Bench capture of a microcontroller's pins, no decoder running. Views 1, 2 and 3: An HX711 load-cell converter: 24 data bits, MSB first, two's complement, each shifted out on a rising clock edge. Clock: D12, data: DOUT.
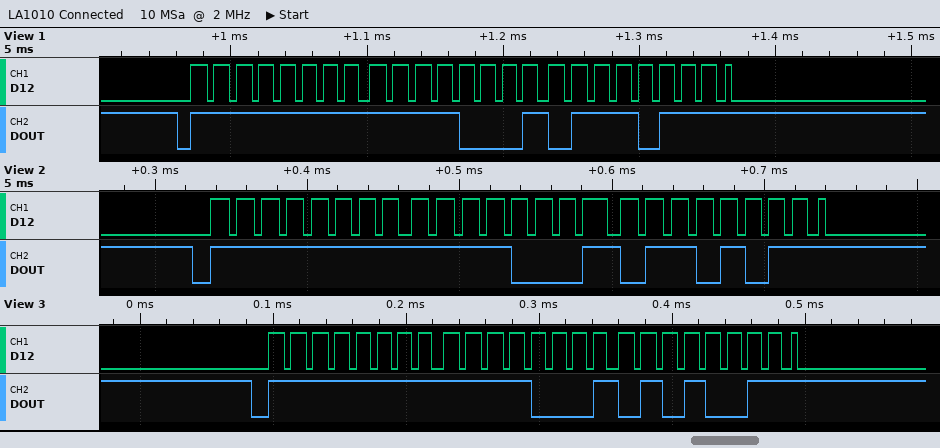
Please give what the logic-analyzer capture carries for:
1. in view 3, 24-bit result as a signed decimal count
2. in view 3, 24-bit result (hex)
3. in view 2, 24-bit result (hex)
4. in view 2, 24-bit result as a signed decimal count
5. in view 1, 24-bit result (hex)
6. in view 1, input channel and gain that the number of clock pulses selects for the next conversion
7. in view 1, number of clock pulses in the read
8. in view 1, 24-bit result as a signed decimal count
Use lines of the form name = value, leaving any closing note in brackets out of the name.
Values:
in view 3, 24-bit result as a signed decimal count = -3757
in view 3, 24-bit result = 0xFFF153
in view 2, 24-bit result = 0xFFF16B
in view 2, 24-bit result as a signed decimal count = -3733
in view 1, 24-bit result = 0xFFF177
in view 1, input channel and gain that the number of clock pulses selects for the next conversion = channel A, gain 128
in view 1, number of clock pulses in the read = 25
in view 1, 24-bit result as a signed decimal count = -3721
